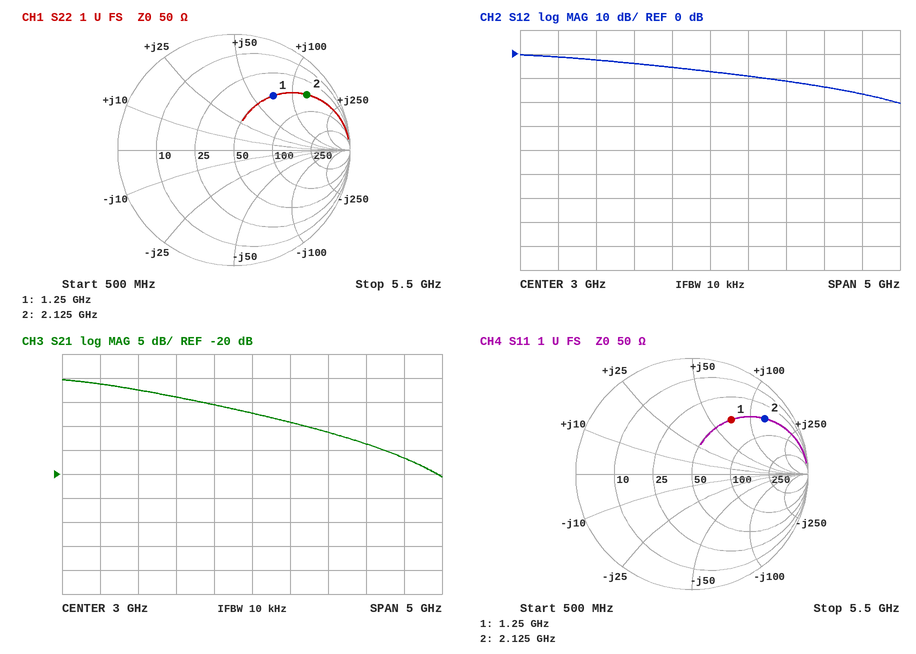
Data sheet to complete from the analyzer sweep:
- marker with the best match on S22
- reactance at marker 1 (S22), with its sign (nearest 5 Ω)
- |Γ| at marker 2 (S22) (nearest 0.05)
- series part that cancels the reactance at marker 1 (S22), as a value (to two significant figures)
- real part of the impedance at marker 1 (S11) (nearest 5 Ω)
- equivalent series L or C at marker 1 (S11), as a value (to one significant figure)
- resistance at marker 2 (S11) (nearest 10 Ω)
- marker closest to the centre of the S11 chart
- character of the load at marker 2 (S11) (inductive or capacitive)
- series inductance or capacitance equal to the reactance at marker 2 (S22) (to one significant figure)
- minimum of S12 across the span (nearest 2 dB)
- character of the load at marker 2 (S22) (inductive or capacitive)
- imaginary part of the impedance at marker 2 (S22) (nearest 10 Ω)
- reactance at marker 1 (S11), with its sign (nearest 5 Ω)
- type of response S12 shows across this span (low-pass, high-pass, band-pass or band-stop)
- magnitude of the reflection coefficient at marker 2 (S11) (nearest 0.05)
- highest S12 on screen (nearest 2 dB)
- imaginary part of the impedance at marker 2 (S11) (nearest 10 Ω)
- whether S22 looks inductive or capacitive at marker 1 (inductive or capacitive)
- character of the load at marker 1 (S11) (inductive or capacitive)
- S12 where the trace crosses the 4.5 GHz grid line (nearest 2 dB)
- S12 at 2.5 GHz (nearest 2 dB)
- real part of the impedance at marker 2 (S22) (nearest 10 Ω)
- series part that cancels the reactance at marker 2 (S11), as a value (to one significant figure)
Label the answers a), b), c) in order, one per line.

a) marker 1
b) +70 Ω
c) 0.80
d) 1.8 pF
e) 50 Ω
f) 9 nH
g) 50 Ω
h) marker 1
i) inductive
j) 10 nH
k) -20 dB
l) inductive
m) +130 Ω
n) +70 Ω
o) low-pass
p) 0.80
q) 0 dB
r) +130 Ω
s) inductive
t) inductive
u) -14 dB
v) -6 dB
w) 50 Ω
x) 600 fF
